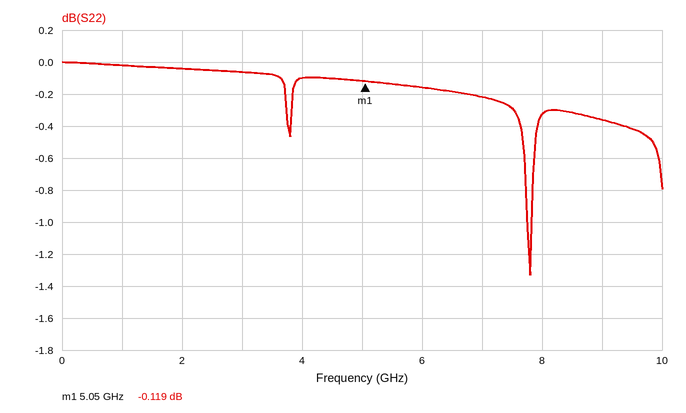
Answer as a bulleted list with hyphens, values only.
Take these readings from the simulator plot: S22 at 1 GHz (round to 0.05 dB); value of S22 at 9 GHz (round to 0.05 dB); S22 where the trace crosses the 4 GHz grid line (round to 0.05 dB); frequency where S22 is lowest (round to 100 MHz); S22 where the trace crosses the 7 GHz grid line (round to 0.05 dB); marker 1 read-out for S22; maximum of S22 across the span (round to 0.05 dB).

- 0.00 dB
- -0.35 dB
- -0.10 dB
- 7.8 GHz
- -0.20 dB
- -0.119 dB
- 0.00 dB
